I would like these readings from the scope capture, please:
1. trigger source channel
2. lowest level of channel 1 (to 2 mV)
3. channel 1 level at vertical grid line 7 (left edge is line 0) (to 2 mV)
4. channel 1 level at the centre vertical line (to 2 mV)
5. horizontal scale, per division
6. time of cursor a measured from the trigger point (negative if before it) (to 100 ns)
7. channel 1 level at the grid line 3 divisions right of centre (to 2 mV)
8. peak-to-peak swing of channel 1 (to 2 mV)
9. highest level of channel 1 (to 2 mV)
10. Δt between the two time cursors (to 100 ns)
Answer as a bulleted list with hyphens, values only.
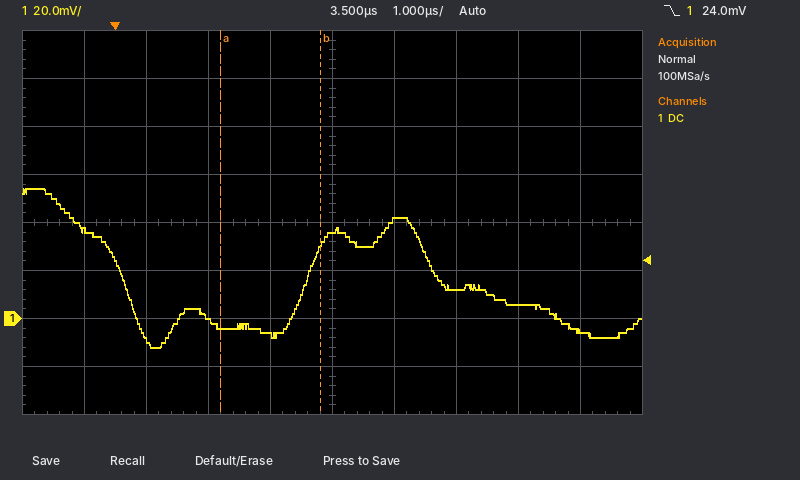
- channel 1
- -12 mV
- 12 mV
- 36 mV
- 1 µs
- +1.7 µs
- 6 mV
- 66 mV
- 54 mV
- 1.6 µs
